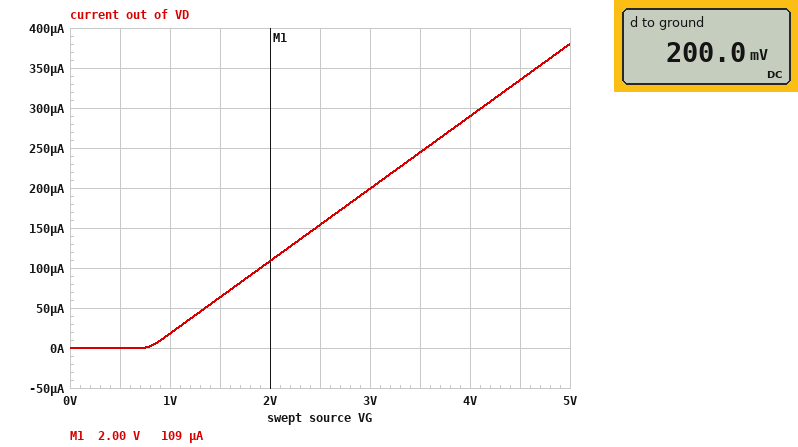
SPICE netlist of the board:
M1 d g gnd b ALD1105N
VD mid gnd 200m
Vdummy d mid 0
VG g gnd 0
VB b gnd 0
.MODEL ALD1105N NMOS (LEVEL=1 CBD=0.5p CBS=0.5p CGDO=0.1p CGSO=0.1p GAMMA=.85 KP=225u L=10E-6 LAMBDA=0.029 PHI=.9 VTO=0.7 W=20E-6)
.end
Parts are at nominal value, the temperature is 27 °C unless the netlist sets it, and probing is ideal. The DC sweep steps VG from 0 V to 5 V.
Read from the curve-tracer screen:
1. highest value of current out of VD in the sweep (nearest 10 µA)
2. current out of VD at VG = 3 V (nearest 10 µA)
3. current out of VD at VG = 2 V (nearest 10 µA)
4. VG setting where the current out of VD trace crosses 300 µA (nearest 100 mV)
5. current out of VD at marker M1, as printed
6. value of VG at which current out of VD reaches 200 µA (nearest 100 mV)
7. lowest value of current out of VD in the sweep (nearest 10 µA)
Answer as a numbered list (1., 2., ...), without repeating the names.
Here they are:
1. 380 µA
2. 200 µA
3. 110 µA
4. 4.1 V
5. 109 µA
6. 3.0 V
7. 0 A
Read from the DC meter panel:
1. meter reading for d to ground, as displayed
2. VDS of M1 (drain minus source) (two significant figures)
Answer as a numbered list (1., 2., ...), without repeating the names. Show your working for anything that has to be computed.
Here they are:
1. 200.0 mV
2. 200 mV = 200 mV
